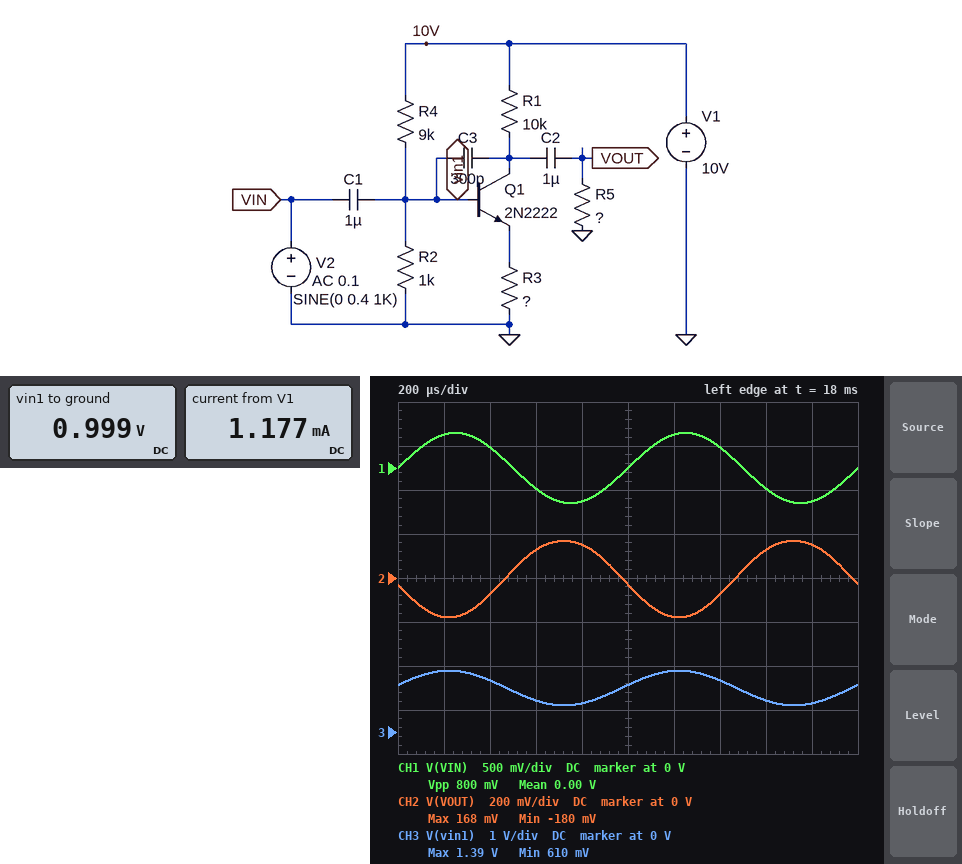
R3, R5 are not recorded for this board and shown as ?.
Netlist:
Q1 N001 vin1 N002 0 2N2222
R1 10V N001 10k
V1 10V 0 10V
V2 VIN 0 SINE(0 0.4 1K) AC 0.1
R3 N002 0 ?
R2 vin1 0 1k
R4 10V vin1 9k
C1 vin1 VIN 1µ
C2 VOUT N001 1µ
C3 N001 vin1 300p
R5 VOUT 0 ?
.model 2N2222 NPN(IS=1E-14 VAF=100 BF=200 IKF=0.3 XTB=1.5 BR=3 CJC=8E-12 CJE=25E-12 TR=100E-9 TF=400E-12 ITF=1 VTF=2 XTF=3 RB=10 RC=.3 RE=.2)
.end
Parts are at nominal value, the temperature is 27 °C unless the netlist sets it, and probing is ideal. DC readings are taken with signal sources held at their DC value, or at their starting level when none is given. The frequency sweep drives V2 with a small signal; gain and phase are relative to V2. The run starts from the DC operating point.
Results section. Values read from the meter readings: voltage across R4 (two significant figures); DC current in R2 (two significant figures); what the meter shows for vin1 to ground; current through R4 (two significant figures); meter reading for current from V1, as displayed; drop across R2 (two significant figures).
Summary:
9.0 V
1.0 mA
0.999 V
1.0 mA
1.177 mA
1.0 V
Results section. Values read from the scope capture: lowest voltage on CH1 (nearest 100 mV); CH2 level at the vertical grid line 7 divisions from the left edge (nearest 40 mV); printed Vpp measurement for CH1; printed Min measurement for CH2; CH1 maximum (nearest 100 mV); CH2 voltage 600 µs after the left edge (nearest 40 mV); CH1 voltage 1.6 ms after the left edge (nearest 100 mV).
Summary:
-400 mV
-80 mV
800 mV
-180 mV
400 mV
120 mV
-200 mV
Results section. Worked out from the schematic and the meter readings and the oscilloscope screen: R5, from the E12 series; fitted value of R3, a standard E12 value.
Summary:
1.2 kΩ
2.2 kΩ
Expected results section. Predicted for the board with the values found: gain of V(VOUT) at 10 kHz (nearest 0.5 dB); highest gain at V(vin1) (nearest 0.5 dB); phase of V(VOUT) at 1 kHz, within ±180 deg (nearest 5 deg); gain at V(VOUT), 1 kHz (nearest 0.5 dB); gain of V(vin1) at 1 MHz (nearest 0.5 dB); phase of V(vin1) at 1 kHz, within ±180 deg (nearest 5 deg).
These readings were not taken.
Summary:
-7.0 dB
0 dB
-170 deg
-7.0 dB
0 dB
10 deg
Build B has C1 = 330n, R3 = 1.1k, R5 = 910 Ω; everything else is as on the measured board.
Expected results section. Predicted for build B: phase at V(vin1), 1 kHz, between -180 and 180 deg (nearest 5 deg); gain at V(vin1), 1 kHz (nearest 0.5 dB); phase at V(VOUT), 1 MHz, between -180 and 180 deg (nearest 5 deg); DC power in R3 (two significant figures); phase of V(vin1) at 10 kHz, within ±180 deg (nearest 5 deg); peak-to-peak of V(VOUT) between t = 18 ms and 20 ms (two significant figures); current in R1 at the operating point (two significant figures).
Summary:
30 deg
-1.0 dB
55 deg
130 µW
5 deg
480 mV
340 µA
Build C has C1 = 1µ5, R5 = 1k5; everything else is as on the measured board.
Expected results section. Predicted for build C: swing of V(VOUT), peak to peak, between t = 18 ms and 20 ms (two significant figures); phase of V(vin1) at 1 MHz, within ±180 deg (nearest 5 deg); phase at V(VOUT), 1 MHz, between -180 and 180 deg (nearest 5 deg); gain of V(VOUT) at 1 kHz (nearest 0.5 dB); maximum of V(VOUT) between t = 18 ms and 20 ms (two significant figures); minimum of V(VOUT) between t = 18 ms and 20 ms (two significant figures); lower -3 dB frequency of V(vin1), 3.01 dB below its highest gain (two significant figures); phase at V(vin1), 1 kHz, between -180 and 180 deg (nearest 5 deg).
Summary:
430 mV
0 deg
35 deg
-5.0 dB
210 mV
-220 mV
120 Hz
5 deg
